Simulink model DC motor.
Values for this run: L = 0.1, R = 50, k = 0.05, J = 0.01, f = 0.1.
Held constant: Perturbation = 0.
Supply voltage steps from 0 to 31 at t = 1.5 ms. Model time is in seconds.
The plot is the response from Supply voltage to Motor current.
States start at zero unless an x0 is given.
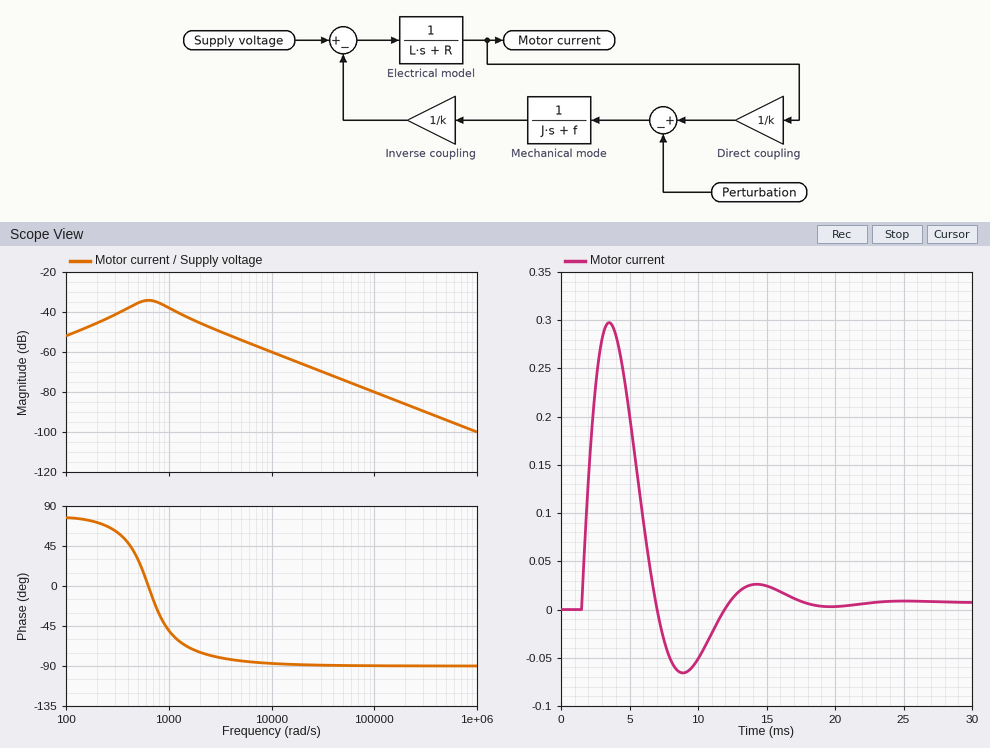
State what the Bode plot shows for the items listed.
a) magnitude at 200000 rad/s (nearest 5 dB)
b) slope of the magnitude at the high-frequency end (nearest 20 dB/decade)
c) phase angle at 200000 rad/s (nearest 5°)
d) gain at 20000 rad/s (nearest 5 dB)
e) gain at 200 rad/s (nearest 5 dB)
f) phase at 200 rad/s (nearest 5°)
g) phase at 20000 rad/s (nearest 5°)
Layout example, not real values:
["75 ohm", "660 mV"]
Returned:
["-85 dB", "-20 dB/decade", "-90°", "-65 dB", "-45 dB", "70°", "-90°"]
